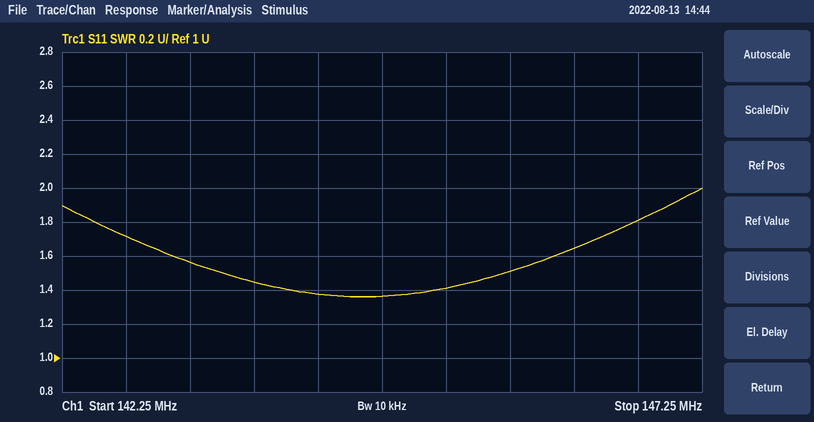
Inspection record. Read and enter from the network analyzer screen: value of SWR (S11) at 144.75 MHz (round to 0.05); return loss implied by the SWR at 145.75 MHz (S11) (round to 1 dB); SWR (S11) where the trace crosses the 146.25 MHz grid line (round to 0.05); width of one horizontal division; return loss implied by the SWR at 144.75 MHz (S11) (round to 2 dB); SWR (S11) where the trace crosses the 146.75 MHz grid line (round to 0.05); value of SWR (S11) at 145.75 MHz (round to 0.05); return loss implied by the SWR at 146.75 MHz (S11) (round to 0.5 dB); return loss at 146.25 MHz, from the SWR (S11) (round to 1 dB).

1.35
14 dB
1.65
500 kHz
16 dB
1.80
1.50
11.0 dB
12 dB
